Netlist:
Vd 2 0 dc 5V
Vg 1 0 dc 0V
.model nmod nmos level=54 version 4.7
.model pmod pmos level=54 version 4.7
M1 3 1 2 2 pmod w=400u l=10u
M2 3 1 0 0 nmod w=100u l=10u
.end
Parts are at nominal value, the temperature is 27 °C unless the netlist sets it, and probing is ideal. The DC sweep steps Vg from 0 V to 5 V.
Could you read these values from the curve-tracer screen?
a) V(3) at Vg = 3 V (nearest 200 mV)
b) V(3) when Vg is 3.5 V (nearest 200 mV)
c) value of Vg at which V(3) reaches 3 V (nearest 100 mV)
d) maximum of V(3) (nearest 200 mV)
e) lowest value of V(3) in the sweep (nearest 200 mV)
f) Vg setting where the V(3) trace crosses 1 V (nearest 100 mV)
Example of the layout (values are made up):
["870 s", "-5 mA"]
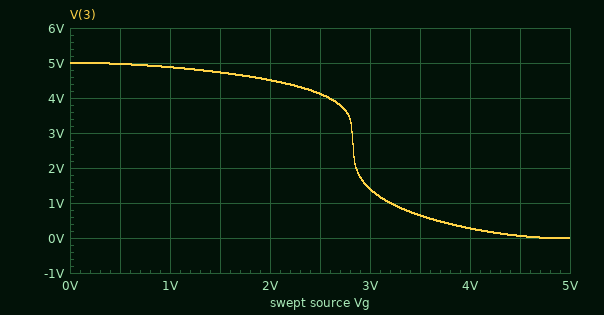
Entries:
["1.4 V", "600 mV", "2.8 V", "5.0 V", "0 V", "3.2 V"]
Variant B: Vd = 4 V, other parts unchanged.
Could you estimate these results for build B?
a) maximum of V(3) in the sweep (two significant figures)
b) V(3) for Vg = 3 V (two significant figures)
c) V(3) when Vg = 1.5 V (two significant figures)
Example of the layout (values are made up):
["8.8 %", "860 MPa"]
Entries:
["4.0 V", "300 mV", "3.7 V"]
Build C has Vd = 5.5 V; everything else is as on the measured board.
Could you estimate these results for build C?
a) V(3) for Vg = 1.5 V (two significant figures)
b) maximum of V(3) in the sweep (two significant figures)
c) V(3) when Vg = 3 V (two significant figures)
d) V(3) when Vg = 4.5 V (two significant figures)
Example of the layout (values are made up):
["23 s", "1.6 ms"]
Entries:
["5.2 V", "5.5 V", "4.1 V", "280 mV"]
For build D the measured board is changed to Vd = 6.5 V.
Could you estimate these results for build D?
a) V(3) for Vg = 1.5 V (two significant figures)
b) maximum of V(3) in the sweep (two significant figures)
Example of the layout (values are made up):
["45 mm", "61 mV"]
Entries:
["6.2 V", "6.5 V"]
